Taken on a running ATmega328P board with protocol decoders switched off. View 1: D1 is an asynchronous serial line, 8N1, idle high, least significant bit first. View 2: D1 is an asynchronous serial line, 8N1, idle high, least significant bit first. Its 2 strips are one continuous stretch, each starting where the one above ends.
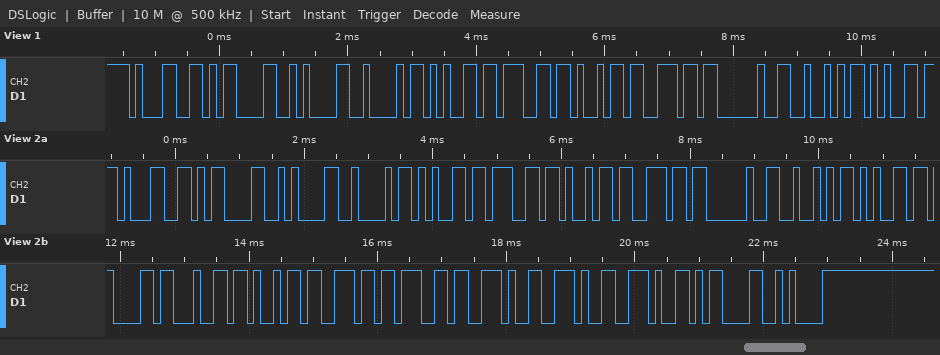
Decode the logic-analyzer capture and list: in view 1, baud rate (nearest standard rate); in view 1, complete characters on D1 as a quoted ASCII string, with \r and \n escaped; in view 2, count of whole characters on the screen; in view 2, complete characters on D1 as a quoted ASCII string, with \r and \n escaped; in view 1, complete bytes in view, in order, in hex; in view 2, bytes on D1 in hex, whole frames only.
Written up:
9600 baud
"1\r\nBegin Re"
21
"1\r\nBegin Reading...\r\n"
0x31 0x0D 0x0A 0x42 0x65 0x67 0x69 0x6E 0x20 0x52 0x65
31 0D 0A 42 65 67 69 6E 20 52 65 61 64 69 6E 67 2E 2E 2E 0D 0A
